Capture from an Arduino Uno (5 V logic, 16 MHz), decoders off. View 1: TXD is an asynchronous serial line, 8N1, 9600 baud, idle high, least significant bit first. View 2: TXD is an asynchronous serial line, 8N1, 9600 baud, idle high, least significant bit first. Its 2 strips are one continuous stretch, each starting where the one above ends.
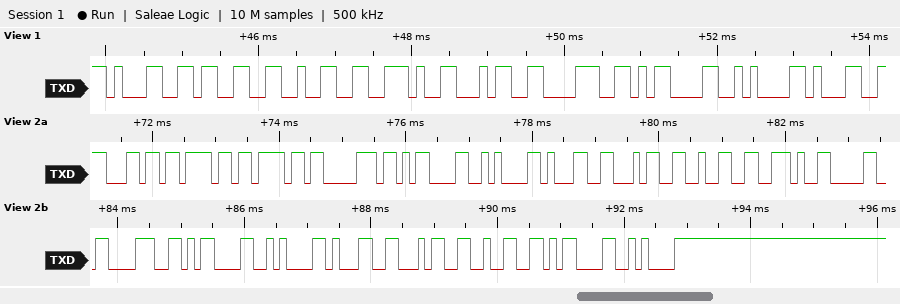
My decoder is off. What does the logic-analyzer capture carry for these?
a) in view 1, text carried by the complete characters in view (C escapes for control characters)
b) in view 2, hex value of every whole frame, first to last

"132.48\r\n1"
6C 6F 6F 70 0D 0A 31 34 32 2E 30 38 0D 0A 31 34 32 0D 0A
